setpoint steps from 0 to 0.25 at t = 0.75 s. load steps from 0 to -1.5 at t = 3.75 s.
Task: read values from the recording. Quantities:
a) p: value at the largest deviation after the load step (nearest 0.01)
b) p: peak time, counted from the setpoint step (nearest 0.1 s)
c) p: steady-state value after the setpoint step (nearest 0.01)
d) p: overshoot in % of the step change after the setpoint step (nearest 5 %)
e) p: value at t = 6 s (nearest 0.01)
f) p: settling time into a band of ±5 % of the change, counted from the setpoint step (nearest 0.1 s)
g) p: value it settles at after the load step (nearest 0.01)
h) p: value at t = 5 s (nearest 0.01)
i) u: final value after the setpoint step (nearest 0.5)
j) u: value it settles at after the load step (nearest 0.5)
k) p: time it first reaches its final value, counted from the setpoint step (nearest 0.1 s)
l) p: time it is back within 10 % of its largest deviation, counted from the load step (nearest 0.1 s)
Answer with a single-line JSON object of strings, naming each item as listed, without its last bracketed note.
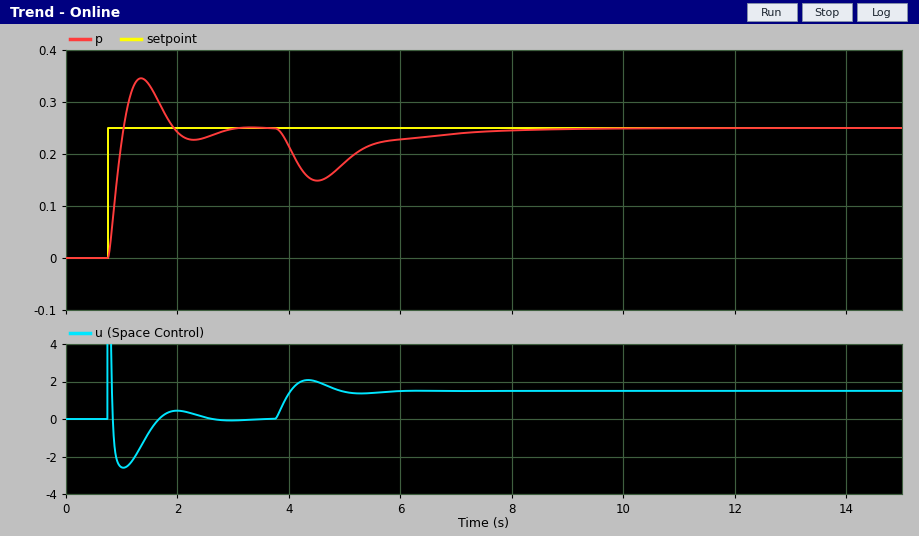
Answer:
{"p: value at the largest deviation after the load step": "0.15", "p: peak time, counted from the setpoint step": "0.6 s", "p: steady-state value after the setpoint step": "0.25", "p: overshoot in % of the step change after the setpoint step": "40 %", "p: value at t = 6 s": "0.23", "p: settling time into a band of ±5 % of the change, counted from the setpoint step": "1.9 s", "p: value it settles at after the load step": "0.25", "p: value at t = 5 s": "0.18", "u: final value after the setpoint step": "0.0", "u: value it settles at after the load step": "1.5", "p: time it first reaches its final value, counted from the setpoint step": "0.3 s", "p: time it is back within 10 % of its largest deviation, counted from the load step": "3.3 s"}
